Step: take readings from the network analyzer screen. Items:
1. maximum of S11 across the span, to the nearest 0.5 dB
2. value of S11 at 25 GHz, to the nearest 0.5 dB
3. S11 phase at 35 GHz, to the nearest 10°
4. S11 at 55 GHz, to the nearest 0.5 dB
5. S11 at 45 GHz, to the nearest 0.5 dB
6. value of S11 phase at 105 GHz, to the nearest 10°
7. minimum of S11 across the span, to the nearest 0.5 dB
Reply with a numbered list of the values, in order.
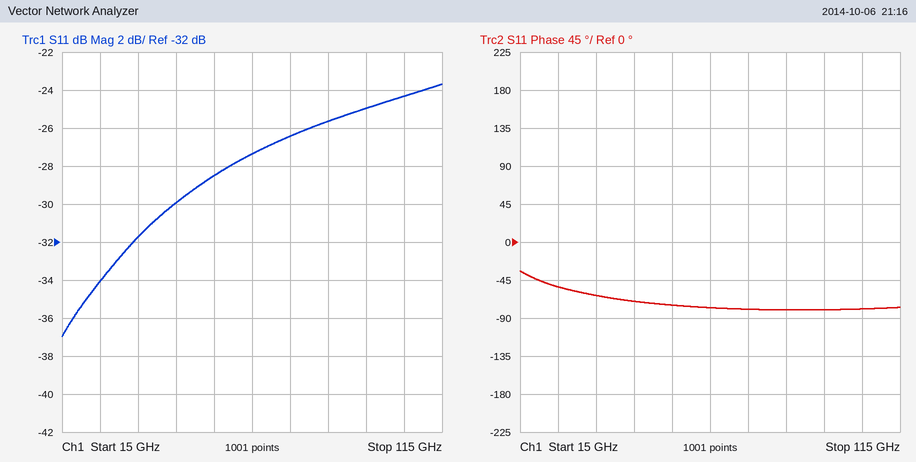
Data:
1. -23.5 dB
2. -34.0 dB
3. -60°
4. -28.5 dB
5. -30.0 dB
6. -80°
7. -37.0 dB
